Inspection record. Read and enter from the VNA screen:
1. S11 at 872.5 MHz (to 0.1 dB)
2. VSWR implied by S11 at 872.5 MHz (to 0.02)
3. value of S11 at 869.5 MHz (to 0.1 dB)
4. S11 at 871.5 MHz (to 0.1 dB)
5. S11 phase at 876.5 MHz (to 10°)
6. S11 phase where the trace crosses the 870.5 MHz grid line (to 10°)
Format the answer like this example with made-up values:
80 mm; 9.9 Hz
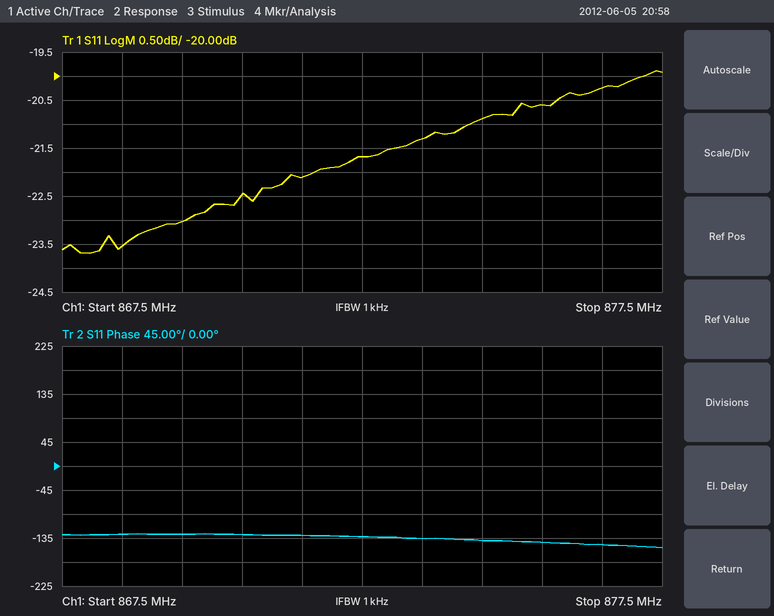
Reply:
-21.7 dB; 1.18; -23.0 dB; -22.1 dB; -150°; -130°
